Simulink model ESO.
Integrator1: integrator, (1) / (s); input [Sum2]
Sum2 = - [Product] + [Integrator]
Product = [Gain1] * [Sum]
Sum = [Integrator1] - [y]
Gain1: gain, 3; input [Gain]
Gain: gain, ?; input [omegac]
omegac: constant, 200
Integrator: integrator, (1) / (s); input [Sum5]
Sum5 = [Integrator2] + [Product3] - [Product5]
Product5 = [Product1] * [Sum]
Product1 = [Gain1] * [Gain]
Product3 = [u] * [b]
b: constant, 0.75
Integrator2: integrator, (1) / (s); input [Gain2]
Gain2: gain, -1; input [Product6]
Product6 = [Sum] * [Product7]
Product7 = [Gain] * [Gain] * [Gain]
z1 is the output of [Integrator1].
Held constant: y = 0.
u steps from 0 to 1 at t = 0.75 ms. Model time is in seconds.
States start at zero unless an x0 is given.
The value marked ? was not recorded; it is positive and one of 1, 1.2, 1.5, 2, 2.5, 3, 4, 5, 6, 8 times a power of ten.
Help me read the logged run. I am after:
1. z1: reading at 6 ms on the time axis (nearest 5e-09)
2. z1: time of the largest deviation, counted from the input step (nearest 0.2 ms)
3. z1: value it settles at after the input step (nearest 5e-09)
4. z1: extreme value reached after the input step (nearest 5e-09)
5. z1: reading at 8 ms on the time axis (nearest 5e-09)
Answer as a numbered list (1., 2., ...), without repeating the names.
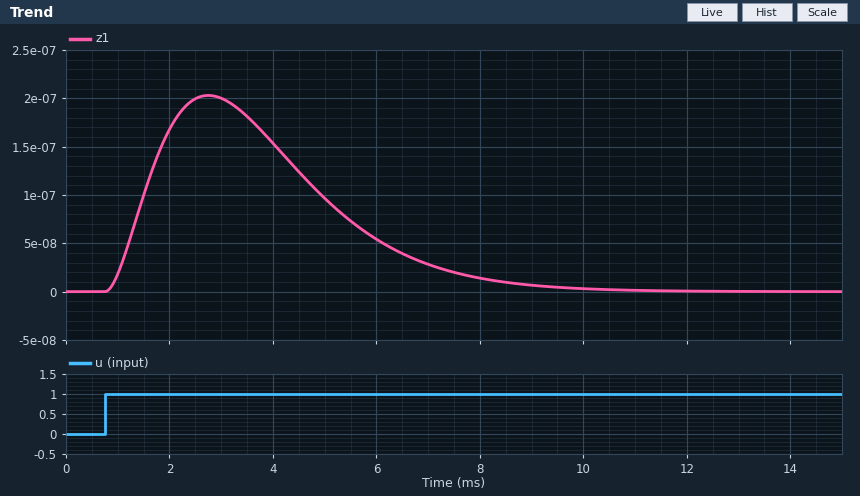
1. 0.000000055
2. 2.0 ms
3. 0.000000000
4. 0.000000205
5. 0.000000015
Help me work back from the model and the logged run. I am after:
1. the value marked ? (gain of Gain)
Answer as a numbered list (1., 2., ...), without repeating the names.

1. 5
